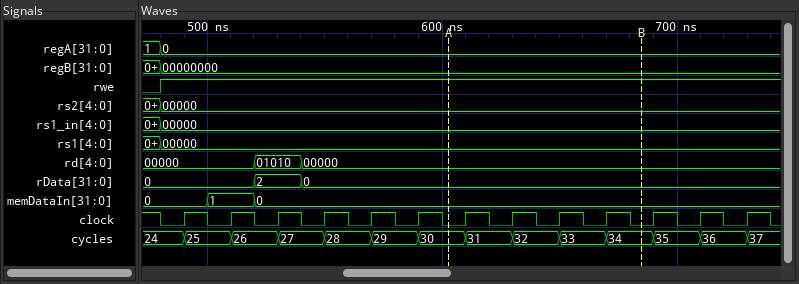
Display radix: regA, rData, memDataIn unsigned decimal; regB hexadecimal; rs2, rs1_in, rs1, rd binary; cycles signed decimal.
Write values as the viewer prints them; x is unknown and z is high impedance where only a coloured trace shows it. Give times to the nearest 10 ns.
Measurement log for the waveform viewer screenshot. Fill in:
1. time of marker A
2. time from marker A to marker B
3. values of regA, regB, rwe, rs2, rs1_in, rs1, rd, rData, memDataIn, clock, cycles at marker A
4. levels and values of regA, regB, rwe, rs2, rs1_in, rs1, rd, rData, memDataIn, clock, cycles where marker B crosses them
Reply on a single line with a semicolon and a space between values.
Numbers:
600 ns; 80 ns; regA=0, regB=00000000, rwe=1, rs2=00000, rs1_in=00000, rs1=00000, rd=00000, rData=0, memDataIn=0, clock=0, cycles=30; regA=0, regB=00000000, rwe=1, rs2=00000, rs1_in=00000, rs1=00000, rd=00000, rData=0, memDataIn=0, clock=0, cycles=34
